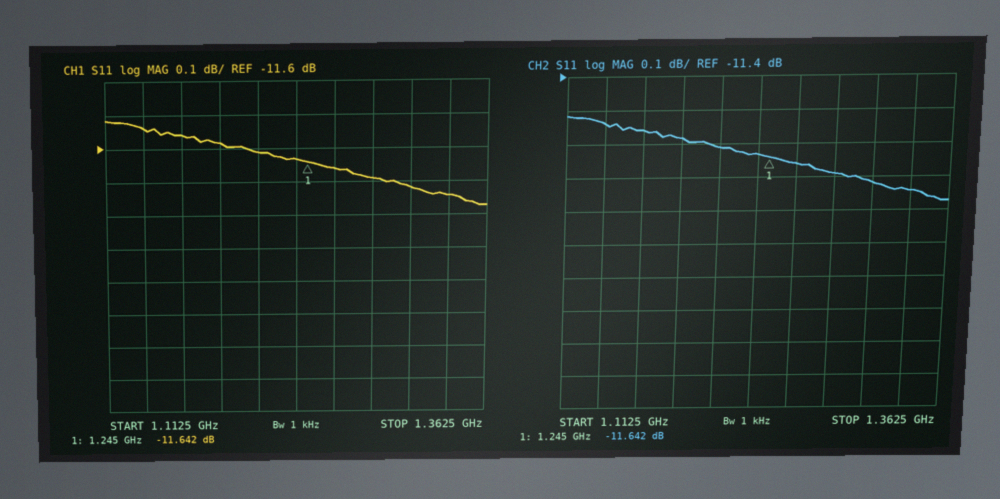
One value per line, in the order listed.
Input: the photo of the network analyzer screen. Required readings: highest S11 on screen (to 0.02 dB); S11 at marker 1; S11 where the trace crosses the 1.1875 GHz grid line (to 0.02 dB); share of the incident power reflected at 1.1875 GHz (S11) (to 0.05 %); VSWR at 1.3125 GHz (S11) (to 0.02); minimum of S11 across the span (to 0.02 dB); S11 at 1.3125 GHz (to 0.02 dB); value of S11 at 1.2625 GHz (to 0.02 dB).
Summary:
-11.52 dB
-11.642 dB
-11.58 dB
6.95 %
1.70
-11.78 dB
-11.72 dB
-11.66 dB
